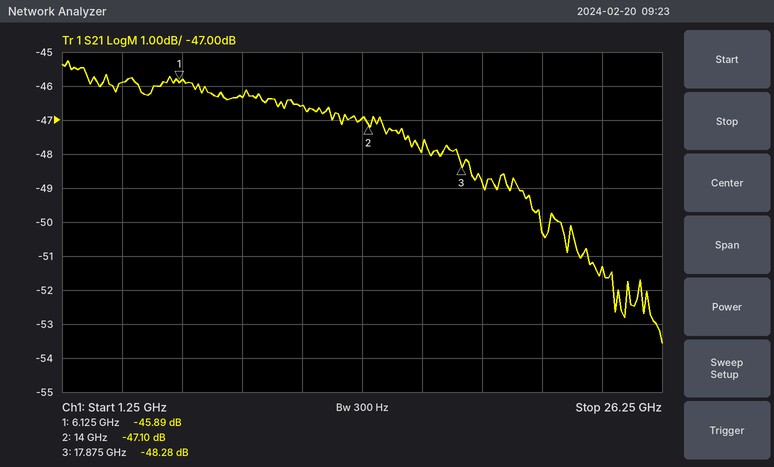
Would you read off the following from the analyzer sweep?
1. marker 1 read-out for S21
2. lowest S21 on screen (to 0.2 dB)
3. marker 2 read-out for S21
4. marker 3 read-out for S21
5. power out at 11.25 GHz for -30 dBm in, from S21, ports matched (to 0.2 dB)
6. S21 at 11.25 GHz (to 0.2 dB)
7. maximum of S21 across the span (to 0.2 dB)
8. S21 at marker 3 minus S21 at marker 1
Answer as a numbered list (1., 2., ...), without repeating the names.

1. -45.89 dB
2. -53.6 dB
3. -47.10 dB
4. -48.28 dB
5. -76.6 dBm
6. -46.6 dB
7. -45.2 dB
8. -2.39 dB
